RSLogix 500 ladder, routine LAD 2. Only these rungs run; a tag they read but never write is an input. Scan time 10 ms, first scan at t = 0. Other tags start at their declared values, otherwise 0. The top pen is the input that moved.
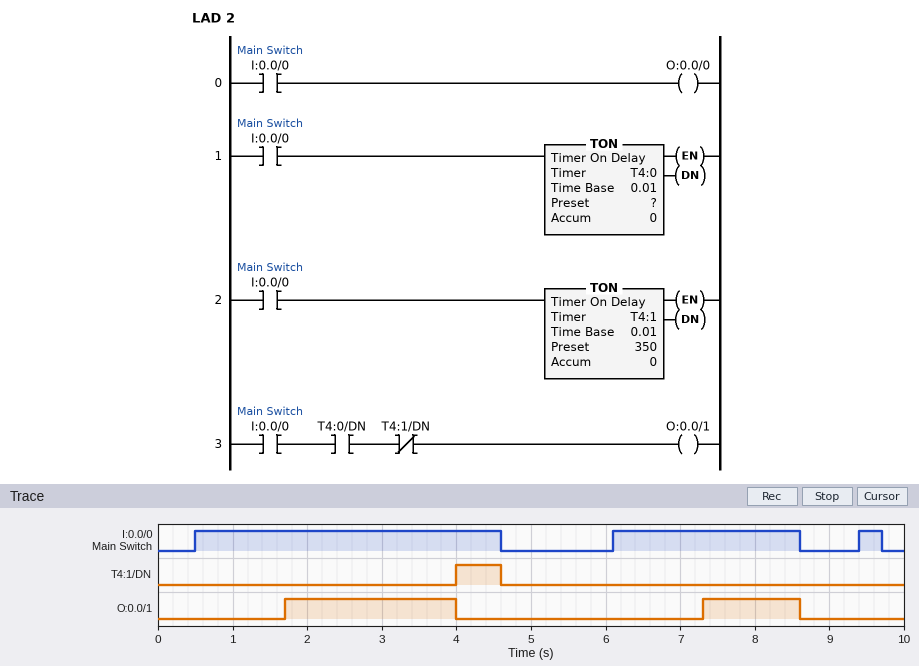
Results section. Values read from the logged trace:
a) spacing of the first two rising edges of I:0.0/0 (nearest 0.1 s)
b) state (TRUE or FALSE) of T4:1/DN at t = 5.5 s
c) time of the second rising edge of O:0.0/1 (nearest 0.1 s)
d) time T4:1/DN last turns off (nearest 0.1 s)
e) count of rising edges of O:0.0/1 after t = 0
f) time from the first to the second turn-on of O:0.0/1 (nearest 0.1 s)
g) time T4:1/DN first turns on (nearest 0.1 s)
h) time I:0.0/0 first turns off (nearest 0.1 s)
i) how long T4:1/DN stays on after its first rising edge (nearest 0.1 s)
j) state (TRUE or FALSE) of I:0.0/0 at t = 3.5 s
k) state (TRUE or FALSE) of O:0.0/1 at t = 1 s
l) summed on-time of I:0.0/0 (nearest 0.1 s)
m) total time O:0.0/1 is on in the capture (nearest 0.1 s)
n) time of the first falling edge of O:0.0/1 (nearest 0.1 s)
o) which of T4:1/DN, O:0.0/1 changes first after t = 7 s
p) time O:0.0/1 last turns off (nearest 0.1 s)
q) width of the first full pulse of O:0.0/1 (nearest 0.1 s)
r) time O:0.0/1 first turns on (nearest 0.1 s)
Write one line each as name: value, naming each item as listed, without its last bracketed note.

spacing of the first two rising edges of I:0.0/0: 5.6 s
state (TRUE or FALSE) of T4:1/DN at t = 5.5 s: FALSE
time of the second rising edge of O:0.0/1: 7.3 s
time T4:1/DN last turns off: 4.6 s
count of rising edges of O:0.0/1 after t = 0: 2
time from the first to the second turn-on of O:0.0/1: 5.6 s
time T4:1/DN first turns on: 4.0 s
time I:0.0/0 first turns off: 4.6 s
how long T4:1/DN stays on after its first rising edge: 0.6 s
state (TRUE or FALSE) of I:0.0/0 at t = 3.5 s: TRUE
state (TRUE or FALSE) of O:0.0/1 at t = 1 s: FALSE
summed on-time of I:0.0/0: 6.9 s
total time O:0.0/1 is on in the capture: 3.6 s
time of the first falling edge of O:0.0/1: 4.0 s
which of T4:1/DN, O:0.0/1 changes first after t = 7 s: O:0.0/1
time O:0.0/1 last turns off: 8.6 s
width of the first full pulse of O:0.0/1: 2.3 s
time O:0.0/1 first turns on: 1.7 s
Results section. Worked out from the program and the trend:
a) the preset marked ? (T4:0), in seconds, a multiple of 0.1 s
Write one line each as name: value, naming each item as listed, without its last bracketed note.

the preset marked ? (T4:0), in seconds, a multiple of 0.1 s: 1.2 s
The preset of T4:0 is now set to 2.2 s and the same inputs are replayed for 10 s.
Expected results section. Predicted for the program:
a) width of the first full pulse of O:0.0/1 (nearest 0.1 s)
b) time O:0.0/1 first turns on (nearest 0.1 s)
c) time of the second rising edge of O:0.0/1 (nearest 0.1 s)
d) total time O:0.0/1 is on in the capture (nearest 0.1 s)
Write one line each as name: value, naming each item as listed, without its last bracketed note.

width of the first full pulse of O:0.0/1: 1.3 s
time O:0.0/1 first turns on: 2.7 s
time of the second rising edge of O:0.0/1: 8.3 s
total time O:0.0/1 is on in the capture: 1.6 s
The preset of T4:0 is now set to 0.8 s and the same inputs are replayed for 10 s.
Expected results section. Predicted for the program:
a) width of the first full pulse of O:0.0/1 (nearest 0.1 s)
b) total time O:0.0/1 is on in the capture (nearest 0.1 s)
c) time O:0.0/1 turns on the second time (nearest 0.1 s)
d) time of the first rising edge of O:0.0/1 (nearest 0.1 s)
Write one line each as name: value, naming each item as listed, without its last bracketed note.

width of the first full pulse of O:0.0/1: 2.7 s
total time O:0.0/1 is on in the capture: 4.4 s
time O:0.0/1 turns on the second time: 6.9 s
time of the first rising edge of O:0.0/1: 1.3 s
